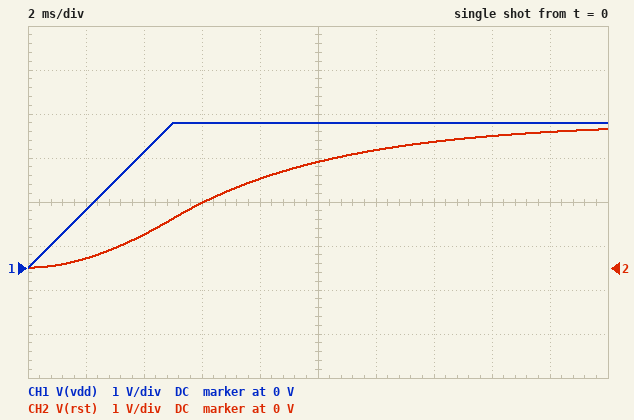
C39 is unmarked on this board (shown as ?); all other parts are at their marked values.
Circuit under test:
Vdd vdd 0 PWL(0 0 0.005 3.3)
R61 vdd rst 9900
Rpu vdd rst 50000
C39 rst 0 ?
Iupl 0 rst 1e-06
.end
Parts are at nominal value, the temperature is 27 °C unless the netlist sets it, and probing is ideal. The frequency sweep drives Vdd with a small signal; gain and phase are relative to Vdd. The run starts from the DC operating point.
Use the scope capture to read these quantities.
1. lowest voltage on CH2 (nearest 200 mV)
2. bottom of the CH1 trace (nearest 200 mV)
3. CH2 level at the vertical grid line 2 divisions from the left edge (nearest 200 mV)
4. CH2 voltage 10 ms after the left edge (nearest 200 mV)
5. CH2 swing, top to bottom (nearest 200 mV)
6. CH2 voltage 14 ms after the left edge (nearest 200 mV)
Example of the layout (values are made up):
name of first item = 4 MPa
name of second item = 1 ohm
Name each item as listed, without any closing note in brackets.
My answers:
lowest voltage on CH2 = 0 V
bottom of the CH1 trace = 0 V
CH2 level at the vertical grid line 2 divisions from the left edge = 800 mV
CH2 voltage 10 ms after the left edge = 2.4 V
CH2 swing, top to bottom = 3.2 V
CH2 voltage 14 ms after the left edge = 2.8 V
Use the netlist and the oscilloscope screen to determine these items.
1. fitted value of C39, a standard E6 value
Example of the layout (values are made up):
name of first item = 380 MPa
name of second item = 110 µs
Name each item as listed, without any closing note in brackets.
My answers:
fitted value of C39, a standard E6 value = 680 nF
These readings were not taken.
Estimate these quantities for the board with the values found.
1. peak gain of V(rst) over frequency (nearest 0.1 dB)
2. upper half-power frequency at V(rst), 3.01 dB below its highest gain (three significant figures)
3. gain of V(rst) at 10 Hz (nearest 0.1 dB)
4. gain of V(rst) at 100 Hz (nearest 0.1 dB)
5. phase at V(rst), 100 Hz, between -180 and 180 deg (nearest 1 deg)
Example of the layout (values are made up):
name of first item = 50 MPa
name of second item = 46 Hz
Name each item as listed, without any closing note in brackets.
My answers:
peak gain of V(rst) over frequency = 0 dB
upper half-power frequency at V(rst), 3.01 dB below its highest gain = 28.3 Hz
gain of V(rst) at 10 Hz = -0.5 dB
gain of V(rst) at 100 Hz = -11.3 dB
phase at V(rst), 100 Hz, between -180 and 180 deg = -74 deg
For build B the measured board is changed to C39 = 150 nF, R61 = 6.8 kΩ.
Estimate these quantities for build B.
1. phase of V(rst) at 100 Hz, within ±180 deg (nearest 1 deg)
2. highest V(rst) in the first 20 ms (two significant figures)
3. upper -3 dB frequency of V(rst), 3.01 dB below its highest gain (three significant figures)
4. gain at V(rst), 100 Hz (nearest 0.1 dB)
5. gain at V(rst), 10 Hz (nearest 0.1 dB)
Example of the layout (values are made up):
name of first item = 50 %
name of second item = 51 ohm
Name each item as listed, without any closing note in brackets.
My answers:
phase of V(rst) at 100 Hz, within ±180 deg = -29 deg
highest V(rst) in the first 20 ms = 3.3 V
upper -3 dB frequency of V(rst), 3.01 dB below its highest gain = 177 Hz
gain at V(rst), 100 Hz = -1.2 dB
gain at V(rst), 10 Hz = 0 dB
